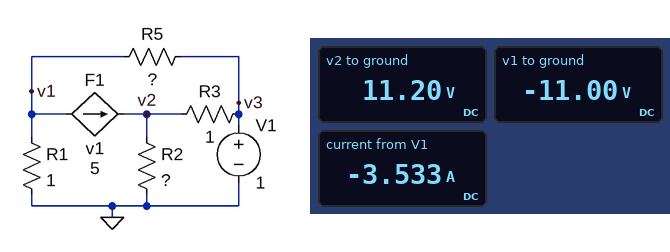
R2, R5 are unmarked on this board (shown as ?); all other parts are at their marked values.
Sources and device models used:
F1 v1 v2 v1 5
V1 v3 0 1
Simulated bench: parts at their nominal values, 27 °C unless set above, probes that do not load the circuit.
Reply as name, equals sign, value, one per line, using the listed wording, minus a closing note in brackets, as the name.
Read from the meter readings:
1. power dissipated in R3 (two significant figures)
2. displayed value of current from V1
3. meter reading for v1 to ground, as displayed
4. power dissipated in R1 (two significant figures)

power dissipated in R3 = 100 W
displayed value of current from V1 = -3.533 A
meter reading for v1 to ground, as displayed = -11.00 V
power dissipated in R1 = 120 W
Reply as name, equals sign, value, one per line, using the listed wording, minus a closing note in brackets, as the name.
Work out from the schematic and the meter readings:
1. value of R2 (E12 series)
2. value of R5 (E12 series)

value of R2 = 1.5 Ω
value of R5 = 1.8 Ω
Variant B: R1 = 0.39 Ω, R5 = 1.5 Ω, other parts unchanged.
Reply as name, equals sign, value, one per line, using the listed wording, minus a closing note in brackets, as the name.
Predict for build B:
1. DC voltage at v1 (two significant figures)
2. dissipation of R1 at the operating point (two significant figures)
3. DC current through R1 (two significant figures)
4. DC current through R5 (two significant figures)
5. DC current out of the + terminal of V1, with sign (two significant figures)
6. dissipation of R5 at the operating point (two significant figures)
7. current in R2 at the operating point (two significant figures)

DC voltage at v1 = -1.3 V
dissipation of R1 at the operating point = 4.2 W
DC current through R1 = 3.3 A
DC current through R5 = 1.5 A
DC current out of the + terminal of V1, with sign = -960 mA
dissipation of R5 at the operating point = 3.5 W
current in R2 at the operating point = 2.3 A
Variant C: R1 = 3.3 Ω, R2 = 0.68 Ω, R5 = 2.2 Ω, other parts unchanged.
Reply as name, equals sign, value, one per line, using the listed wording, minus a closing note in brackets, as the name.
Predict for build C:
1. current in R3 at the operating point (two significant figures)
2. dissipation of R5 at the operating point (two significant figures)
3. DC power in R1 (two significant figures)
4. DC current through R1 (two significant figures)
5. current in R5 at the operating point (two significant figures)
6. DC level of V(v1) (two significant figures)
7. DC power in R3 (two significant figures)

current in R3 at the operating point = 1.4 A
dissipation of R5 at the operating point = 2.2 W
DC power in R1 = 3.1 W
DC current through R1 = 970 mA
current in R5 at the operating point = 1.0 A
DC level of V(v1) = 3.2 V
DC power in R3 = 1.9 W
